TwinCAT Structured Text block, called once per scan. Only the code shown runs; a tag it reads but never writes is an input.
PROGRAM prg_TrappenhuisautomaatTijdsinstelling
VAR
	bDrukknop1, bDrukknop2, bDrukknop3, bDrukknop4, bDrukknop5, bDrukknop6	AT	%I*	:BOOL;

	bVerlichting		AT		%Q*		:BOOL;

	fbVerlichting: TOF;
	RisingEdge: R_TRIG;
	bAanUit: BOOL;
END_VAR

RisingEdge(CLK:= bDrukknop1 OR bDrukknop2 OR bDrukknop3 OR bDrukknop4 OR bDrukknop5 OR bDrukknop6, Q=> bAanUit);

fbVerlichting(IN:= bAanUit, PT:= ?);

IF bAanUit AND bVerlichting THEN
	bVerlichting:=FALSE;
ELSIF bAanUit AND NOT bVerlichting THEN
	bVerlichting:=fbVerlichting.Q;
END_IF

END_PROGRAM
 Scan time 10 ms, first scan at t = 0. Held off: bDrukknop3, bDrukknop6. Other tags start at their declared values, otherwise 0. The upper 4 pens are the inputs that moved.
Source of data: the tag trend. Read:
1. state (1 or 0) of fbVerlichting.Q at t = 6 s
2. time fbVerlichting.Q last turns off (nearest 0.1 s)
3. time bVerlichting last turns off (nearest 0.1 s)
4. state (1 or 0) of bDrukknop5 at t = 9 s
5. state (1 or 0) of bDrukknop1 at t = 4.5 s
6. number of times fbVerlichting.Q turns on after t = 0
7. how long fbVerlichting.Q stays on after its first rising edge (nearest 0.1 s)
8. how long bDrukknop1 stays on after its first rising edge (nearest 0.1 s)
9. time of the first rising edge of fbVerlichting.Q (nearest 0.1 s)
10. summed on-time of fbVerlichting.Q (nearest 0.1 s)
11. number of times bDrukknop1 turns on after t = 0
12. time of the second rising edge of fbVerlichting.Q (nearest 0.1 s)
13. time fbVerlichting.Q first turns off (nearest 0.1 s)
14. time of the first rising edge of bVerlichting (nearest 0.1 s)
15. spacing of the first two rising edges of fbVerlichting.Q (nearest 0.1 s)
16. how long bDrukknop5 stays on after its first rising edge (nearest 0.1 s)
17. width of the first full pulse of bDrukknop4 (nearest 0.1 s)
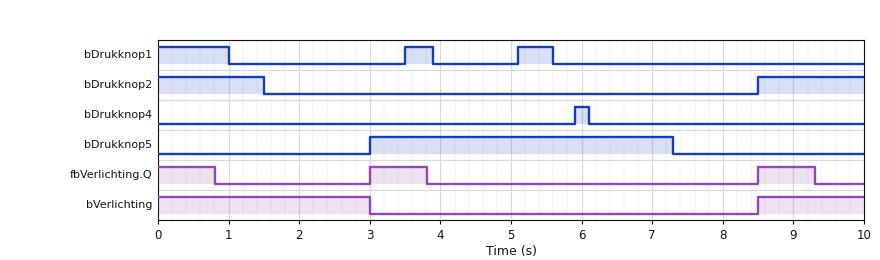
0
9.3 s
3.0 s
0
0
2
0.8 s
0.4 s
3.0 s
2.4 s
2
8.5 s
0.8 s
8.5 s
5.5 s
4.3 s
0.2 s
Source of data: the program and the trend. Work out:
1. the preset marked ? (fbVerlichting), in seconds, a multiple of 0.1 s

0.8 s
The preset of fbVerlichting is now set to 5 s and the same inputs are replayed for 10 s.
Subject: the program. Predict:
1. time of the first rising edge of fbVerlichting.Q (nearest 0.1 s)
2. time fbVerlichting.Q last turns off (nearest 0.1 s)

8.5 s
8.0 s
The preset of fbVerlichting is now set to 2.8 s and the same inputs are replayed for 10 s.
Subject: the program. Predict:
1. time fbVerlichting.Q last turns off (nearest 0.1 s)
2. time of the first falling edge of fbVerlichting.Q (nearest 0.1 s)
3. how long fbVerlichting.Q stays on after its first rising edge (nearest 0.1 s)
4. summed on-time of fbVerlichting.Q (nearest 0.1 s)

5.8 s
2.8 s
2.8 s
7.1 s
